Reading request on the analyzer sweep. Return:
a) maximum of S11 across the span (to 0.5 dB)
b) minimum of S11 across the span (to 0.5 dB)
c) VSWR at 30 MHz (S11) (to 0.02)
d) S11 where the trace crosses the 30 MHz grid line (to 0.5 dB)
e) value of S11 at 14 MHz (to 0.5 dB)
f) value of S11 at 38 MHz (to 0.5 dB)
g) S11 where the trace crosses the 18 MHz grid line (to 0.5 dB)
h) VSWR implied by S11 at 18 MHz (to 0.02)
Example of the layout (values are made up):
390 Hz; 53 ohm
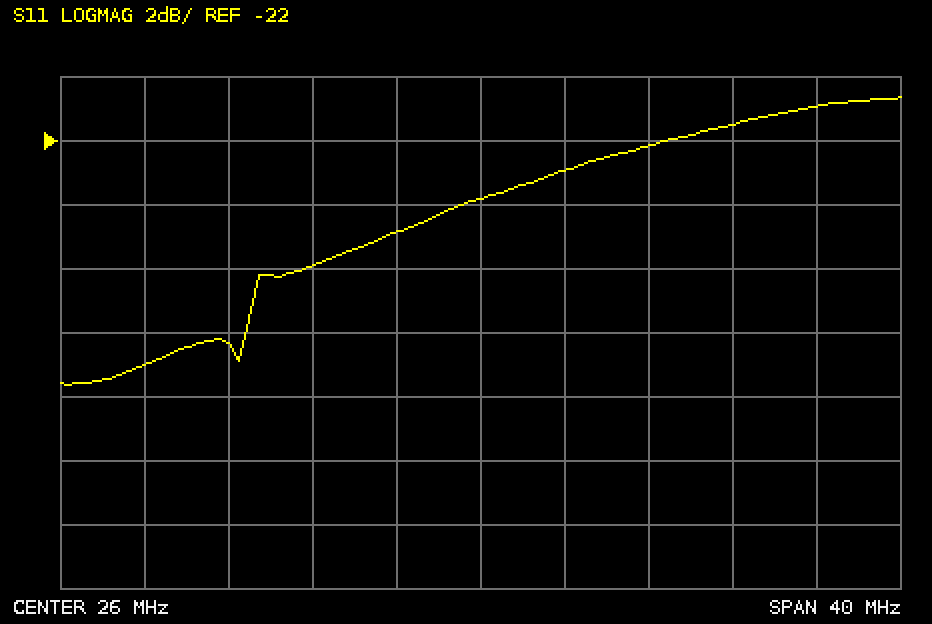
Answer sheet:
-20.5 dB; -29.5 dB; 1.16; -23.0 dB; -28.5 dB; -21.5 dB; -26.0 dB; 1.10
